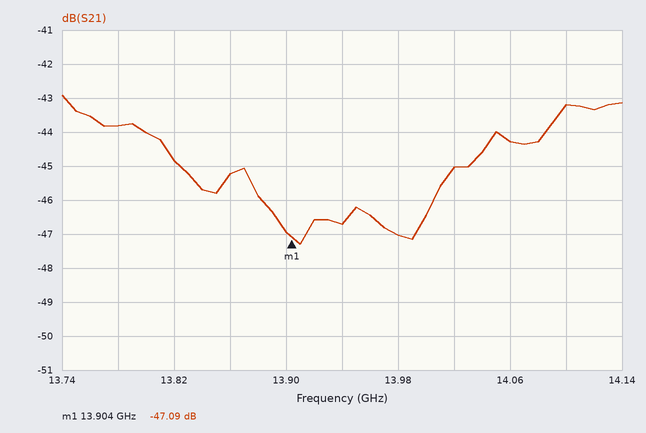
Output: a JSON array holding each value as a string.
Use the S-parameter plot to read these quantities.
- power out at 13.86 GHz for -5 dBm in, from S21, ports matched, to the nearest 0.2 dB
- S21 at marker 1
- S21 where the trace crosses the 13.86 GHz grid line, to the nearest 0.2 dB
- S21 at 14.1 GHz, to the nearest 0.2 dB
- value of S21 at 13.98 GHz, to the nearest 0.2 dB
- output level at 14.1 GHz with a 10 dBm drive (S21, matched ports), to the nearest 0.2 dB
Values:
["-50.2 dBm", "-47.09 dB", "-45.2 dB", "-43.2 dB", "-47.0 dB", "-33.2 dBm"]
